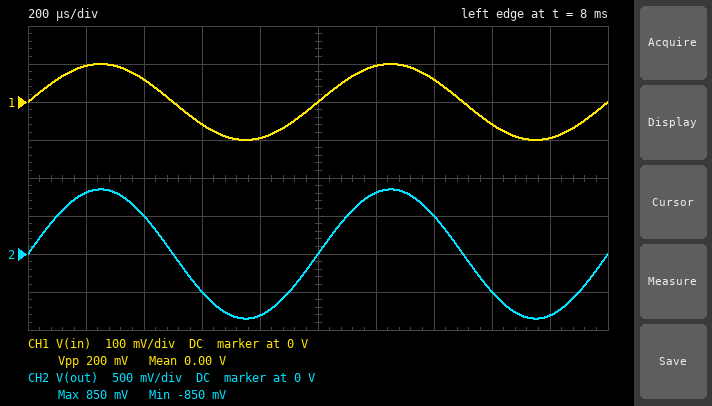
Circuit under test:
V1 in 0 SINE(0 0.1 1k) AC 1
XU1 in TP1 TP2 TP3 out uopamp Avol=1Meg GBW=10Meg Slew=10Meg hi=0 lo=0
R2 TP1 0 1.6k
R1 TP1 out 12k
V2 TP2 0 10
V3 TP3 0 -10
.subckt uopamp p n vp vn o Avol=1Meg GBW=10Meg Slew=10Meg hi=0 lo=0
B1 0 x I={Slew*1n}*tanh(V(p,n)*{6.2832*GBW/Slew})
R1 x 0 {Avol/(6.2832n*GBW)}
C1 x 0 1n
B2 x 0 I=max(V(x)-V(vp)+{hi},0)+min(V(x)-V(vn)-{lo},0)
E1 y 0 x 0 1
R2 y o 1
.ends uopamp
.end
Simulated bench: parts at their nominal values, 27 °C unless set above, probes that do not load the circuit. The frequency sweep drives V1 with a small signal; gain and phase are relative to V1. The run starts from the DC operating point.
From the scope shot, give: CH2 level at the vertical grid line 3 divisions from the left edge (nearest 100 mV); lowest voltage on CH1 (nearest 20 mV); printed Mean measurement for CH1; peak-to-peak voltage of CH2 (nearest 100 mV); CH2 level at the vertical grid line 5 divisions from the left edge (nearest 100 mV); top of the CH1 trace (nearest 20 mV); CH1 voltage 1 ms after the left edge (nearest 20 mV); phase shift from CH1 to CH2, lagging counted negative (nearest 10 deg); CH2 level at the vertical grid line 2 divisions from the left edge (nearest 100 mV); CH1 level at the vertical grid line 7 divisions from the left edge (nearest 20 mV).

-500 mV
-100 mV
0.00 V
1.7 V
0 V
100 mV
0 V
0 deg
500 mV
60 mV
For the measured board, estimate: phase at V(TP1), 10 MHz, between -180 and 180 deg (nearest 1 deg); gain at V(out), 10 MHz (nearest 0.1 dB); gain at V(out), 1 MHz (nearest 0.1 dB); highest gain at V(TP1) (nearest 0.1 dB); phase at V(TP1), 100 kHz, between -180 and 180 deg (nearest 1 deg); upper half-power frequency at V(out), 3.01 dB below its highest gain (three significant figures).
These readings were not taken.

-83 deg
-0.1 dB
16.2 dB
0 dB
-5 deg
1.18 MHz
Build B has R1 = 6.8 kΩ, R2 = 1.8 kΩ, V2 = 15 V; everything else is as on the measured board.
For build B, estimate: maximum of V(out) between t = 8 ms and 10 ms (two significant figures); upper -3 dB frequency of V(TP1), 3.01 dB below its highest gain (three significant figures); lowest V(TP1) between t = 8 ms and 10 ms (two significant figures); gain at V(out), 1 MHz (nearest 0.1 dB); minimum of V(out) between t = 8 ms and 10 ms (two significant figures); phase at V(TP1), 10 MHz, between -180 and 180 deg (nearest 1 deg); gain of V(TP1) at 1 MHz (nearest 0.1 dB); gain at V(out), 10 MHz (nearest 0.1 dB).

480 mV
2.09 MHz
-100 mV
12.7 dB
-480 mV
-78 deg
-0.9 dB
-0.2 dB
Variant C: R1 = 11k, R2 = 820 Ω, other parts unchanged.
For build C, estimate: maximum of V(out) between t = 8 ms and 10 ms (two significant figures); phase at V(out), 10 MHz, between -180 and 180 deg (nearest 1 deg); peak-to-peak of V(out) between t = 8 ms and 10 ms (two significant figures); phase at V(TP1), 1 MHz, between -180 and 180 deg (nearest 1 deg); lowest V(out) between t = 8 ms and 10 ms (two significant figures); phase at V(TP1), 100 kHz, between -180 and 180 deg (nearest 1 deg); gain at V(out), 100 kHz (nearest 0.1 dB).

1.4 V
-86 deg
2.9 V
-55 deg
-1.4 V
-8 deg
23.1 dB
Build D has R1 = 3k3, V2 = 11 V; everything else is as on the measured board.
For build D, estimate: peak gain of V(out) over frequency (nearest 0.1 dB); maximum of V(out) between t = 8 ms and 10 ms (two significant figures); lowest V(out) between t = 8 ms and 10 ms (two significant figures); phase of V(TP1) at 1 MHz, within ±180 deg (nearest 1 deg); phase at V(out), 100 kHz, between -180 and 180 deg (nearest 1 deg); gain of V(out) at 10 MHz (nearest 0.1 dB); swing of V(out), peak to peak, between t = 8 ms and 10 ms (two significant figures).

9.7 dB
310 mV
-310 mV
-17 deg
-2 deg
-0.4 dB
610 mV
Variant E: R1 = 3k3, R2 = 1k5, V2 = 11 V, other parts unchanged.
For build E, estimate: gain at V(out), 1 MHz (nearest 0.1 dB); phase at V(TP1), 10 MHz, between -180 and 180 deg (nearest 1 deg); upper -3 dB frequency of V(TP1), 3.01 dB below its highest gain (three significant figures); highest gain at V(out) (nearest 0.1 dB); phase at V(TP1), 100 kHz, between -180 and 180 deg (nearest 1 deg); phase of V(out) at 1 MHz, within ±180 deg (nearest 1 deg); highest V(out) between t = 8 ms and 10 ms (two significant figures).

9.7 dB
-73 deg
3.12 MHz
10.1 dB
-2 deg
-18 deg
320 mV
